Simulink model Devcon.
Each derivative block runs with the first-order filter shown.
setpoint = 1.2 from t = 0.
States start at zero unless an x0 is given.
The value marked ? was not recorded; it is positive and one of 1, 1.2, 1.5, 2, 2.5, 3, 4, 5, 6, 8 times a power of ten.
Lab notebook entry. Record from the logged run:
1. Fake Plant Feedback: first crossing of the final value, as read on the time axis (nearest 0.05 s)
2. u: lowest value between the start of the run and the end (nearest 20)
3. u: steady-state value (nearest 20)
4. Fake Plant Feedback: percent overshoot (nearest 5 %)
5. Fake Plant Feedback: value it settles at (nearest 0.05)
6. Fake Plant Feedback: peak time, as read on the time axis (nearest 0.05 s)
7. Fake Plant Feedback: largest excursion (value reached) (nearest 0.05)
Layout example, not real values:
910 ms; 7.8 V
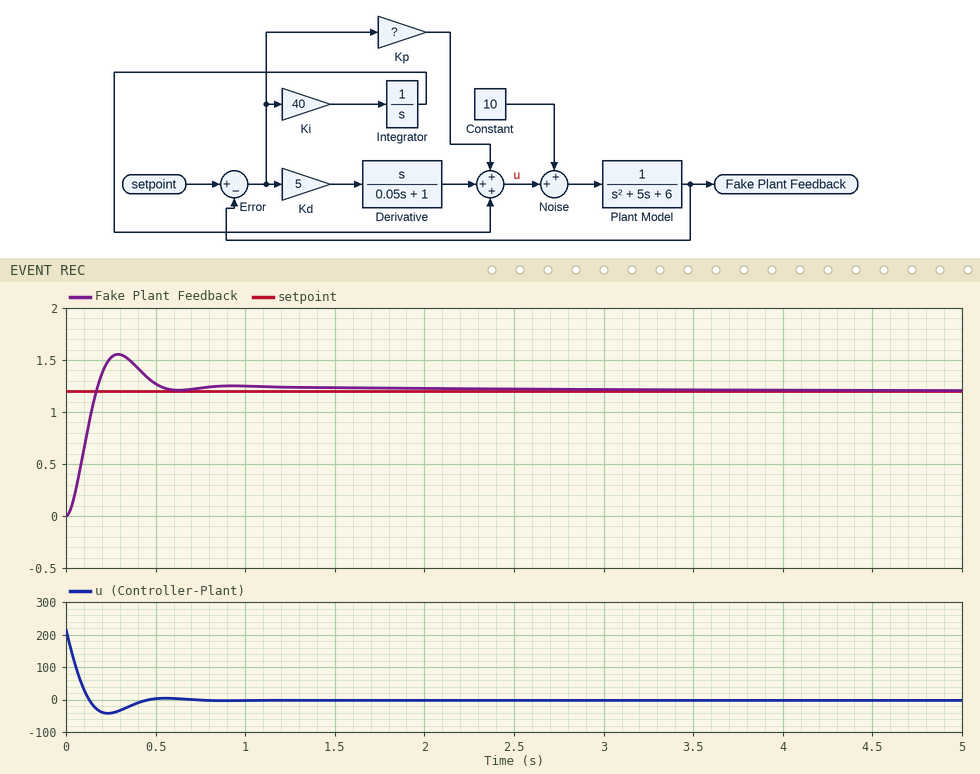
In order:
0.15 s; -40; 0; 30 %; 1.20; 0.30 s; 1.55
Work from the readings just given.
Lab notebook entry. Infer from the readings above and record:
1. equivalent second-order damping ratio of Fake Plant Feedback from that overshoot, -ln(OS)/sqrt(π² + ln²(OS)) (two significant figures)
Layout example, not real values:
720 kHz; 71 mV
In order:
0.36
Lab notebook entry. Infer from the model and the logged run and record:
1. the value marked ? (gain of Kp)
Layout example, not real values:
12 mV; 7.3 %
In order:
80
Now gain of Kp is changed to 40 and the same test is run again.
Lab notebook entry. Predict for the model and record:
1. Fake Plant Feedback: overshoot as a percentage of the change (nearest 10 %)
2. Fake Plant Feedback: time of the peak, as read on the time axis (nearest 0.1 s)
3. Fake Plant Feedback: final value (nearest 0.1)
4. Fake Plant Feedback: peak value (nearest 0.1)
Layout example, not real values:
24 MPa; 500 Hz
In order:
20 %; 0.4 s; 1.2; 1.4
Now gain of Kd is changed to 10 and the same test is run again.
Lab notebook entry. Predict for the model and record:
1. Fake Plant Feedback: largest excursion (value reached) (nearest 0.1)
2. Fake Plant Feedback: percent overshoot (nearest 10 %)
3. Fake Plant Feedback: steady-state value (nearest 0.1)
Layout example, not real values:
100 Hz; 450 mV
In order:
1.4; 20 %; 1.2
